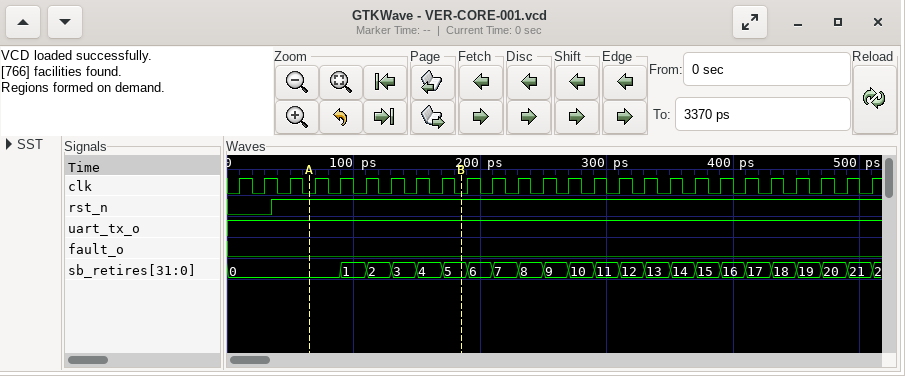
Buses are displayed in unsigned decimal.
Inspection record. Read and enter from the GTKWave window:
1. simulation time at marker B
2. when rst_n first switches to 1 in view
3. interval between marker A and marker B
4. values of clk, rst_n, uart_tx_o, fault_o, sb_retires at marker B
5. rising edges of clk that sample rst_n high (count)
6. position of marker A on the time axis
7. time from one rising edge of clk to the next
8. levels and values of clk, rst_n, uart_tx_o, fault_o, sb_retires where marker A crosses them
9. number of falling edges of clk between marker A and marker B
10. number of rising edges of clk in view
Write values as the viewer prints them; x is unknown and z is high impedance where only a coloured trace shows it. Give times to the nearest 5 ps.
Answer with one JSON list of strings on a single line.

["185 ps", "35 ps", "120 ps", "clk=0, rst_n=1, uart_tx_o=1, fault_o=0, sb_retires=5", "24", "65 ps", "20 ps", "clk=0, rst_n=1, uart_tx_o=1, fault_o=0, sb_retires=0", "6", "26"]
